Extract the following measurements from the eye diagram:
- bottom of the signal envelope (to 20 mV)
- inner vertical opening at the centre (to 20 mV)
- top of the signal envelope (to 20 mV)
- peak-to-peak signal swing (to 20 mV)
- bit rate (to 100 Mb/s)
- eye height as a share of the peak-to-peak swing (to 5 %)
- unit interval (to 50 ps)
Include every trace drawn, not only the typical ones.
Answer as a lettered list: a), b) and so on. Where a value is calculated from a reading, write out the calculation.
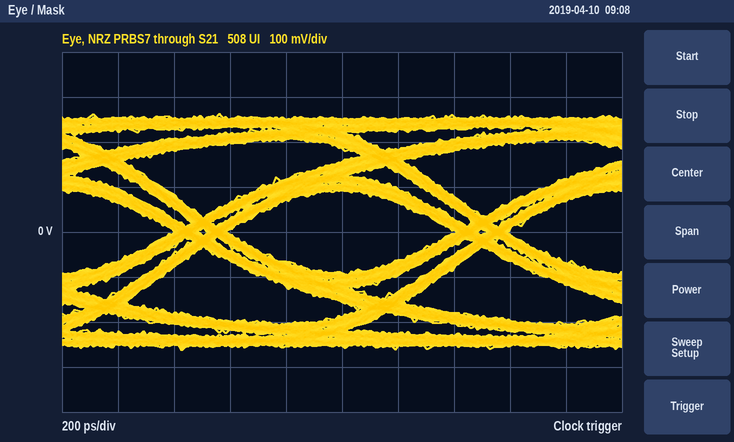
a) -260 mV
b) 180 mV
c) 260 mV
d) 520 mV
e) 1.0 Gb/s
f) 180 mV / 520 mV ≈ 35 %
g) 1.00 ns
